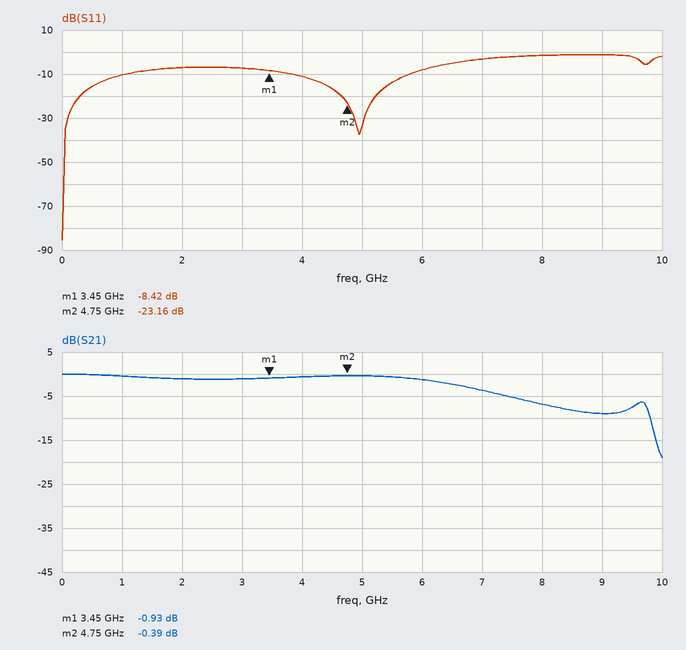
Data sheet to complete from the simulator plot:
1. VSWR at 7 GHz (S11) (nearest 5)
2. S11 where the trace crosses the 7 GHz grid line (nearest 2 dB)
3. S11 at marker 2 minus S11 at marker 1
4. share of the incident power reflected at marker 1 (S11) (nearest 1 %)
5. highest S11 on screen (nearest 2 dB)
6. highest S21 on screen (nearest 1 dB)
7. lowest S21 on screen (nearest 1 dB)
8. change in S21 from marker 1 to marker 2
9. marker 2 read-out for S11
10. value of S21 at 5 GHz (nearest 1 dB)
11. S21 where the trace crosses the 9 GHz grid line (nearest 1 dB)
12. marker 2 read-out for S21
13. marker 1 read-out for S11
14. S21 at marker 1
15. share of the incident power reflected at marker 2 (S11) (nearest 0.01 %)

5
-4 dB
-14.74 dB
14 %
-2 dB
0 dB
-19 dB
0.54 dB
-23.16 dB
0 dB
-9 dB
-0.39 dB
-8.42 dB
-0.93 dB
0.48 %
